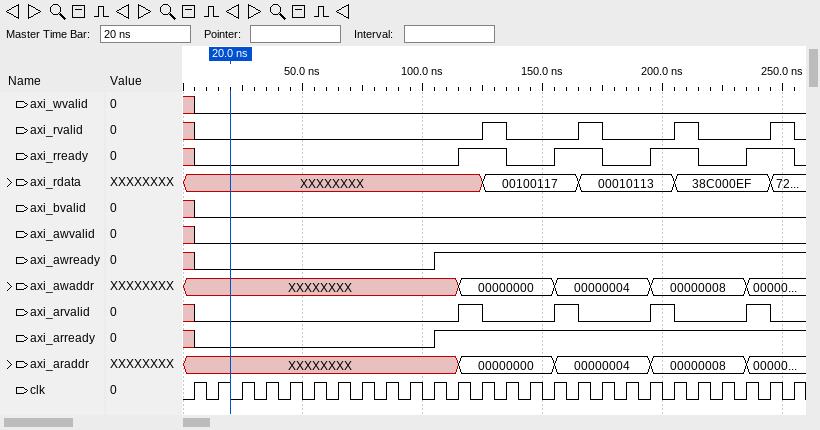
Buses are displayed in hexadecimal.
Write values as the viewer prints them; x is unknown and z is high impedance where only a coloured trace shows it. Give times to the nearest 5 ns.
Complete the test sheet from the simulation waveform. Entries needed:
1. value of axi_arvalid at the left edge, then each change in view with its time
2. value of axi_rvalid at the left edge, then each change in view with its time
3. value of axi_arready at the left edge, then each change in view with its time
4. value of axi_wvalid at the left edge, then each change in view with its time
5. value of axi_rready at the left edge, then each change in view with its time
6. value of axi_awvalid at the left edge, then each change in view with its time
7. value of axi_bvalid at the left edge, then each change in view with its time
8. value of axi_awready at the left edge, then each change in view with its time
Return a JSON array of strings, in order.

["x, 0 at 5 ns, 1 at 115 ns, 0 at 125 ns, 1 at 155 ns, 0 at 165 ns, 1 at 195 ns, 0 at 205 ns, 1 at 235 ns, 0 at 245 ns", "x, 0 at 5 ns, 1 at 125 ns, 0 at 135 ns, 1 at 165 ns, 0 at 175 ns, 1 at 205 ns, 0 at 215 ns, 1 at 245 ns, 0 at 255 ns", "x, 0 at 5 ns, 1 at 105 ns", "x, 0 at 5 ns", "x, 0 at 5 ns, 1 at 115 ns, 0 at 135 ns, 1 at 155 ns, 0 at 175 ns, 1 at 195 ns, 0 at 215 ns, 1 at 235 ns, 0 at 255 ns", "x, 0 at 5 ns", "x, 0 at 5 ns", "x, 0 at 5 ns, 1 at 105 ns"]
